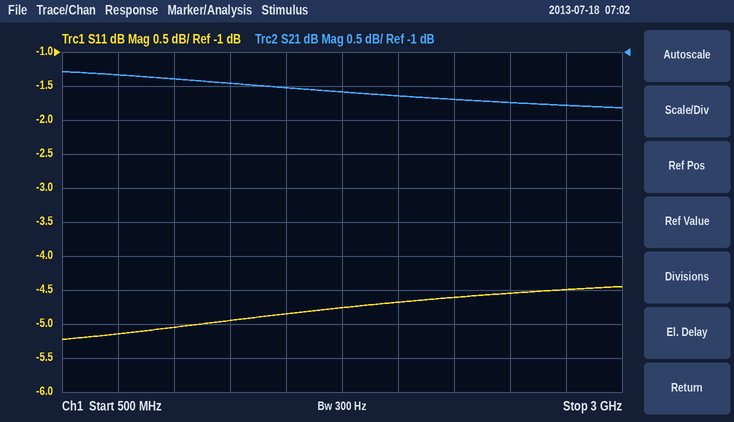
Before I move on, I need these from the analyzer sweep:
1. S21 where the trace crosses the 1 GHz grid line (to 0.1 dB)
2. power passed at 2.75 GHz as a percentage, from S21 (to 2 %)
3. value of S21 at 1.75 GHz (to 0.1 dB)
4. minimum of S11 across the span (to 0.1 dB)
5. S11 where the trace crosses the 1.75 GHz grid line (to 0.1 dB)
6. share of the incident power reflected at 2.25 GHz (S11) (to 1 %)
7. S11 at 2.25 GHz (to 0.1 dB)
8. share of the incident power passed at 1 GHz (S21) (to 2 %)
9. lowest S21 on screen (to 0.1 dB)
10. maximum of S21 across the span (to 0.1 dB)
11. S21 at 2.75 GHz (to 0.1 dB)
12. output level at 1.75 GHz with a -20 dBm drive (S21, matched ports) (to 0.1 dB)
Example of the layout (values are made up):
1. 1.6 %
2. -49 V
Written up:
1. -1.4 dB
2. 66 %
3. -1.6 dB
4. -5.2 dB
5. -4.8 dB
6. 35 %
7. -4.6 dB
8. 72 %
9. -1.8 dB
10. -1.3 dB
11. -1.8 dB
12. -21.6 dBm
